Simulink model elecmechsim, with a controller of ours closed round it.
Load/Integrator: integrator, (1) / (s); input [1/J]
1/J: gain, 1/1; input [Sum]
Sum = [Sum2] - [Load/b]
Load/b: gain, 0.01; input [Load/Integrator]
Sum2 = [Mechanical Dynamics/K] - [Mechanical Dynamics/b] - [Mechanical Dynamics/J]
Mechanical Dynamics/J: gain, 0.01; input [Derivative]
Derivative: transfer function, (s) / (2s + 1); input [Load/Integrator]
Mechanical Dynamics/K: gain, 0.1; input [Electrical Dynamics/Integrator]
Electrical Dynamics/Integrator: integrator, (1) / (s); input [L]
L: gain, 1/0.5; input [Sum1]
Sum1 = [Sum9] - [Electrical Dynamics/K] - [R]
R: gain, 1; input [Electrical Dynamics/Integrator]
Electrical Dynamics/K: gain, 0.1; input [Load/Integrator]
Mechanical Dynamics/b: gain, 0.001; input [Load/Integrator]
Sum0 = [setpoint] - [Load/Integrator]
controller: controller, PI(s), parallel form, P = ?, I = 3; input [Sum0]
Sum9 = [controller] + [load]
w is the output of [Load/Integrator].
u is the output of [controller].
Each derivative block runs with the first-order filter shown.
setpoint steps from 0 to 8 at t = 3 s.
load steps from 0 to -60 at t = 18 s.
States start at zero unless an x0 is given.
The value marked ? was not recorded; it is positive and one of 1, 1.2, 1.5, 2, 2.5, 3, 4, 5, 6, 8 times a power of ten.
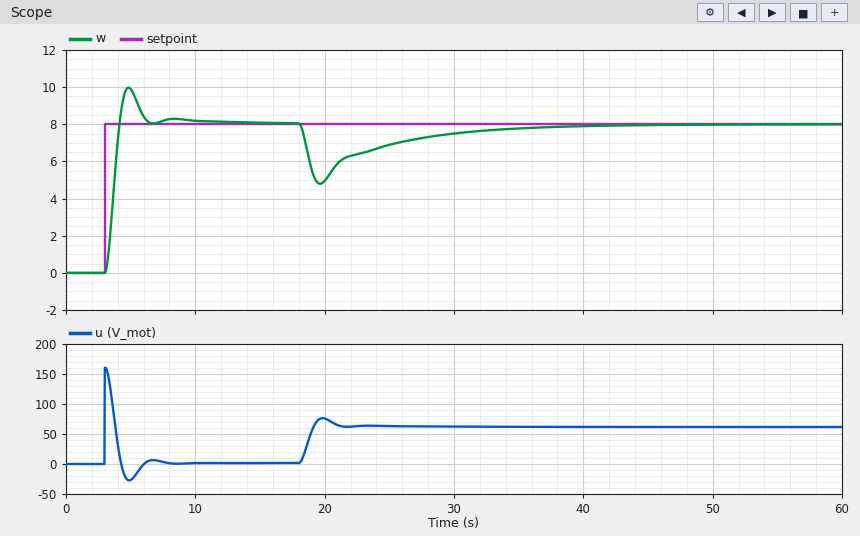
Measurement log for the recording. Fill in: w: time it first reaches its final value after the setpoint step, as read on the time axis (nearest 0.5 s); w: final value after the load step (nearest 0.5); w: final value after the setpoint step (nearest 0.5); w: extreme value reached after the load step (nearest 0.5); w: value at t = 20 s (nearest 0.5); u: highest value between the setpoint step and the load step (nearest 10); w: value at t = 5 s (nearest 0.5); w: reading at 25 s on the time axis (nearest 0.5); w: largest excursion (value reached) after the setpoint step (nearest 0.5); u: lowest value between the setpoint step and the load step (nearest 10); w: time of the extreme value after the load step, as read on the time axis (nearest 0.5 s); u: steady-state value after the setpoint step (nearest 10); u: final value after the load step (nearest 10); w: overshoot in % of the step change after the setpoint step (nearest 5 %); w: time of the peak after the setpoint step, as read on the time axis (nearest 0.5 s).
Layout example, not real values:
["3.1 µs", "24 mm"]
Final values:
["4.0 s", "8.0", "8.0", "5.0", "5.0", "160", "10.0", "7.0", "10.0", "-30", "19.5 s", "0", "60", "25 %", "5.0 s"]
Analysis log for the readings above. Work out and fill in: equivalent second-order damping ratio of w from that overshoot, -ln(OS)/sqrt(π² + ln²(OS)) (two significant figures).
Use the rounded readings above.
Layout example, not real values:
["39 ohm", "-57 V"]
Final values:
["0.40"]
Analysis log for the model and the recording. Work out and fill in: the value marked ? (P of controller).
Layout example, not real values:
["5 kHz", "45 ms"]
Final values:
["20"]
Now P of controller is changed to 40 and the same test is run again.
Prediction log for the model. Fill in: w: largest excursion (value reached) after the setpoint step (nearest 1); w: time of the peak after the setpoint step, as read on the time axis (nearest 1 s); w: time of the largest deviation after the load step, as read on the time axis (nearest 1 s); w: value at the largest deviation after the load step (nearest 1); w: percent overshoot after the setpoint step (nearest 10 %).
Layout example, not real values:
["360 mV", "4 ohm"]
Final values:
["11", "4 s", "19 s", "6", "30 %"]
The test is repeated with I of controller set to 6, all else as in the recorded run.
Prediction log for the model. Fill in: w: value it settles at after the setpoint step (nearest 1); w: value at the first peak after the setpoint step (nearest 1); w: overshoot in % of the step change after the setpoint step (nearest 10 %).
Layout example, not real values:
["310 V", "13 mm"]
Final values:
["8", "11", "30 %"]
